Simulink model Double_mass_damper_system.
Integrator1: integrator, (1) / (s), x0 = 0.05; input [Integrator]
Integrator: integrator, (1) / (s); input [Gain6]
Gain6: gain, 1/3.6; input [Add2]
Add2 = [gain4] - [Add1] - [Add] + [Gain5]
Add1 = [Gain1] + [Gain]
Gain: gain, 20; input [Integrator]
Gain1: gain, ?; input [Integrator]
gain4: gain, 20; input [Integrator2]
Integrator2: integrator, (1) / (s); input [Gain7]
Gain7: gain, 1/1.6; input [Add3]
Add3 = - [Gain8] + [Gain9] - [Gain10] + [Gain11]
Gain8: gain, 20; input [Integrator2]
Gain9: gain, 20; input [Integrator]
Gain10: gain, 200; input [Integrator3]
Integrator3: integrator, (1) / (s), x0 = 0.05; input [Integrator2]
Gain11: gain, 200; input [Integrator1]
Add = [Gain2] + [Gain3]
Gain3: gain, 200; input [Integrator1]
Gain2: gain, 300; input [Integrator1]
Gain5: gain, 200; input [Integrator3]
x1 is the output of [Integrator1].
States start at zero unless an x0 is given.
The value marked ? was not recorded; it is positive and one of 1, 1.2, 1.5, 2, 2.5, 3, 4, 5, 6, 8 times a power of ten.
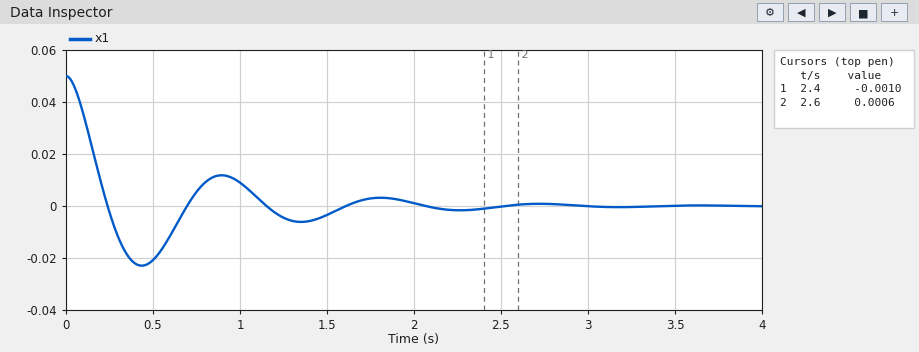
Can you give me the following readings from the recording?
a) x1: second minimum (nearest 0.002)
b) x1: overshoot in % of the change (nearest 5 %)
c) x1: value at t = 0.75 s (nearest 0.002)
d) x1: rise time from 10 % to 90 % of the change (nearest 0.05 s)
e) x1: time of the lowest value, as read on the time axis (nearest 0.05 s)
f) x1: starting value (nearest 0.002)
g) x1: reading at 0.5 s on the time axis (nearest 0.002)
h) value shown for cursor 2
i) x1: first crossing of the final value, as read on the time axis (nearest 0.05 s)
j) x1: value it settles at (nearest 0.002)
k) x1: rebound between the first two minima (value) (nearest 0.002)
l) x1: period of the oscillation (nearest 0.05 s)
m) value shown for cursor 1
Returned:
-0.006
45 %
0.006
0.15 s
0.45 s
0.050
-0.020
0.0006
0.25 s
0.000
0.012
0.90 s
-0.0010
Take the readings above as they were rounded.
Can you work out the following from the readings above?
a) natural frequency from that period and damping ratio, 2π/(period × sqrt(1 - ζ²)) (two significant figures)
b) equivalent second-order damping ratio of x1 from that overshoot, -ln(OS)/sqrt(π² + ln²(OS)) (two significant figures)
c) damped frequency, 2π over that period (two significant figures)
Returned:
7.2 rad/s
0.25
7.0 rad/s
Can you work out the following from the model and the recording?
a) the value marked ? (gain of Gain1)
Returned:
15
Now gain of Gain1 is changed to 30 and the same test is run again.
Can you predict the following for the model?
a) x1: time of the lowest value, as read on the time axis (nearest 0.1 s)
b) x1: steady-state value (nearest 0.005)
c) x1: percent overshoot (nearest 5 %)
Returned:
0.5 s
0.000
25 %
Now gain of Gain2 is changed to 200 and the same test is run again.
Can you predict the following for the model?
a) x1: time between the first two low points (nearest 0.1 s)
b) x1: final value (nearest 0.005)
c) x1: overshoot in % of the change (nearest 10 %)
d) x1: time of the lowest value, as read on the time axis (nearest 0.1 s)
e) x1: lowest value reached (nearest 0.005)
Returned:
1.1 s
0.000
40 %
0.5 s
-0.020
